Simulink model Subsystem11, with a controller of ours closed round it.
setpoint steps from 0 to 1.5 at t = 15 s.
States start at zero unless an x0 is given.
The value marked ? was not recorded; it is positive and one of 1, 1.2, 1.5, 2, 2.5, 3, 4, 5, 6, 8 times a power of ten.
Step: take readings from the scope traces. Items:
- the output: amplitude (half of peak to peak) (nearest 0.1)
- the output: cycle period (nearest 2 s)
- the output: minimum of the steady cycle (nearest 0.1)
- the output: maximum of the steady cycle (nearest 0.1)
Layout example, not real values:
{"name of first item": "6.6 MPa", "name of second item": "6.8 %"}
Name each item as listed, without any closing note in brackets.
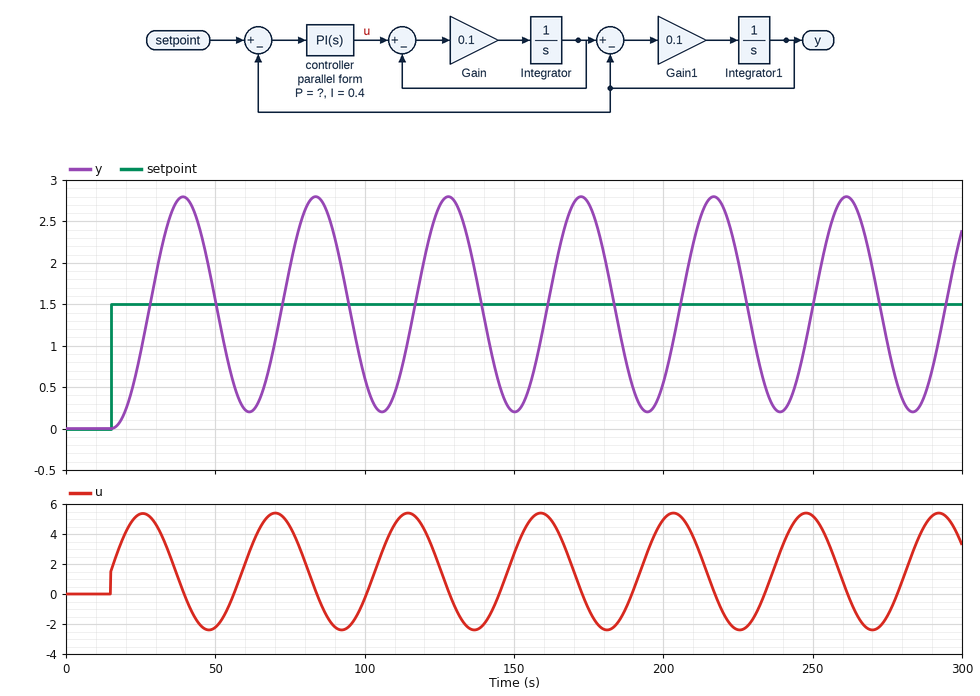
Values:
{"the output: amplitude (half of peak to peak)": "1.3", "the output: cycle period": "44 s", "the output: minimum of the steady cycle": "0.2", "the output: maximum of the steady cycle": "2.8"}
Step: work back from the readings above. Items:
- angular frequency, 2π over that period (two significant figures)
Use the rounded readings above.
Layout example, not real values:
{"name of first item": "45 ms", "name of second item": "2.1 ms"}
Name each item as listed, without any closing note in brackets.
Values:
{"angular frequency, 2π over that period": "0.14 rad/s"}
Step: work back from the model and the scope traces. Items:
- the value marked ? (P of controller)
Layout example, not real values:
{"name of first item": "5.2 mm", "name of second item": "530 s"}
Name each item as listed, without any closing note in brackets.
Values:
{"the value marked ?": "1"}
